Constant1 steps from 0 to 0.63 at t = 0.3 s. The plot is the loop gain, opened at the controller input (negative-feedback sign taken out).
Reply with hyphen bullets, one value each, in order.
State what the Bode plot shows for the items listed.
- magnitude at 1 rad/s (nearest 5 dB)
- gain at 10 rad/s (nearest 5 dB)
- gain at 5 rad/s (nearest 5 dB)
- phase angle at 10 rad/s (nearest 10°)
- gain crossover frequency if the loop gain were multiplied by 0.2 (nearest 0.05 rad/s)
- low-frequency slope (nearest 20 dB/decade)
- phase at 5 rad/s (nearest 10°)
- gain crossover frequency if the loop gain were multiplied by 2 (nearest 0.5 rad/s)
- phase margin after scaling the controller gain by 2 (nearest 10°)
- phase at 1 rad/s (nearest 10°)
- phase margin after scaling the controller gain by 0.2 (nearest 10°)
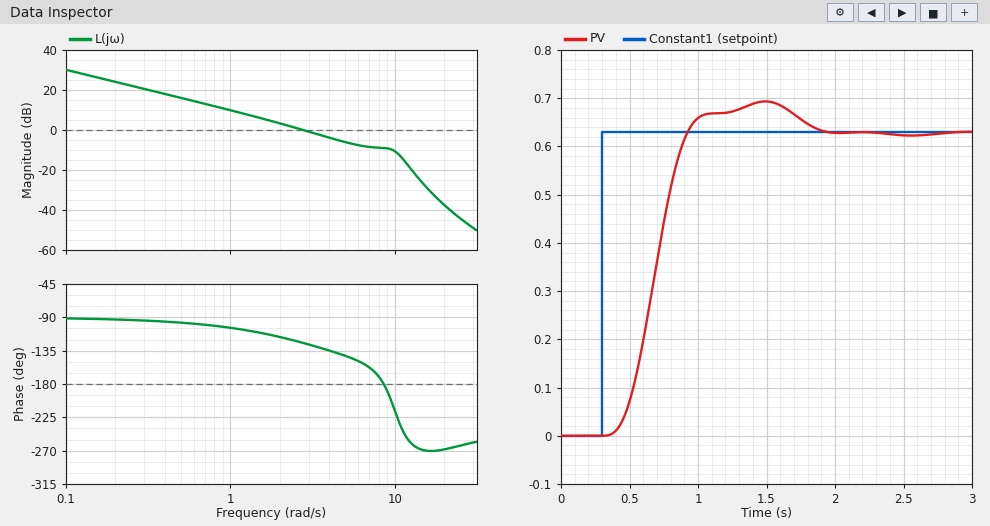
- 10 dB
- -10 dB
- -5 dB
- -220°
- 0.65 rad/s
- -20 dB/decade
- -140°
- 5.0 rad/s
- 40°
- -100°
- 80°
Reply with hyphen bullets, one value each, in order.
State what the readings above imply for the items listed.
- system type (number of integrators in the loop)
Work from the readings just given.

- 1
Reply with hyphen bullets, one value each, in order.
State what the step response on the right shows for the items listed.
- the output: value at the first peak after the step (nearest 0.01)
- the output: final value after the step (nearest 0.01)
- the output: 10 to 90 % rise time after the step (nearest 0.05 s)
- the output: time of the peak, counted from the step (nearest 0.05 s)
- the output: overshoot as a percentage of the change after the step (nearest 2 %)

- 0.69
- 0.63
- 0.35 s
- 1.20 s
- 10 %
